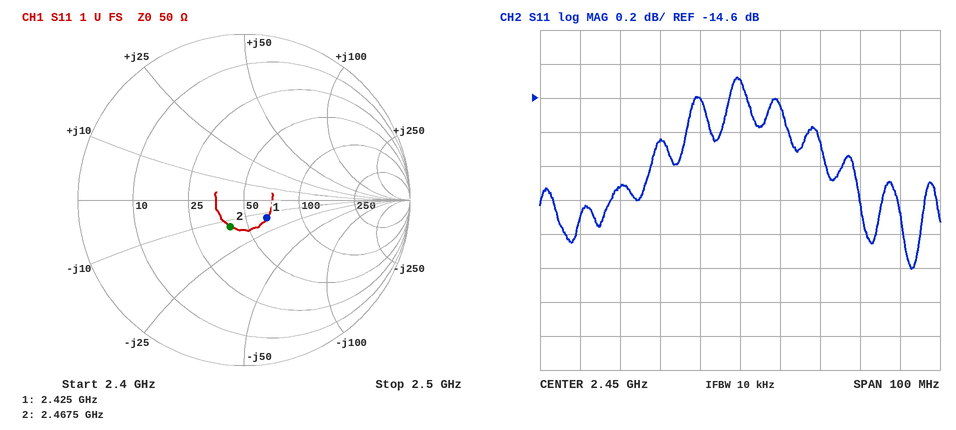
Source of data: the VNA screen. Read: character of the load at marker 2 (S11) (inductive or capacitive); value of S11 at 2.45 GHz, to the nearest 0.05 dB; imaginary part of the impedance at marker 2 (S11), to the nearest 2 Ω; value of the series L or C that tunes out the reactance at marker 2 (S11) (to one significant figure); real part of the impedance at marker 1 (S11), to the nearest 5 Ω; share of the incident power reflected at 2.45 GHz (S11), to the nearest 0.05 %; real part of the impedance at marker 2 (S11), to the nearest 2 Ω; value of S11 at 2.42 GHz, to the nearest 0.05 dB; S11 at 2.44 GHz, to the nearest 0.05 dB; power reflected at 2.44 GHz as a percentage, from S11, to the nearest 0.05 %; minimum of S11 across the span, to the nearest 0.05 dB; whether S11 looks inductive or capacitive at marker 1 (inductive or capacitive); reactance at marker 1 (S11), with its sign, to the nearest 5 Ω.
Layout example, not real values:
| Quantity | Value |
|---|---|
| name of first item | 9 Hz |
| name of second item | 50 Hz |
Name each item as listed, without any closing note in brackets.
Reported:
| Quantity | Value |
|---|---|
| character of the load at marker 2 (S11) | capacitive |
| value of S11 at 2.45 GHz, to the nearest 0.05 dB | -14.50 dB |
| imaginary part of the impedance at marker 2 (S11), to the nearest 2 Ω | -14 Ω |
| value of the series L or C that tunes out the reactance at marker 2 (S11) | 900 pH |
| real part of the impedance at marker 1 (S11), to the nearest 5 Ω | 65 Ω |
| share of the incident power reflected at 2.45 GHz (S11), to the nearest 0.05 % | 3.55 % |
| real part of the impedance at marker 2 (S11), to the nearest 2 Ω | 40 Ω |
| value of S11 at 2.42 GHz, to the nearest 0.05 dB | -15.10 dB |
| S11 at 2.44 GHz, to the nearest 0.05 dB | -14.60 dB |
| power reflected at 2.44 GHz as a percentage, from S11, to the nearest 0.05 % | 3.45 % |
| minimum of S11 across the span, to the nearest 0.05 dB | -15.60 dB |
| whether S11 looks inductive or capacitive at marker 1 | capacitive |
| reactance at marker 1 (S11), with its sign, to the nearest 5 Ω | -15 Ω |
